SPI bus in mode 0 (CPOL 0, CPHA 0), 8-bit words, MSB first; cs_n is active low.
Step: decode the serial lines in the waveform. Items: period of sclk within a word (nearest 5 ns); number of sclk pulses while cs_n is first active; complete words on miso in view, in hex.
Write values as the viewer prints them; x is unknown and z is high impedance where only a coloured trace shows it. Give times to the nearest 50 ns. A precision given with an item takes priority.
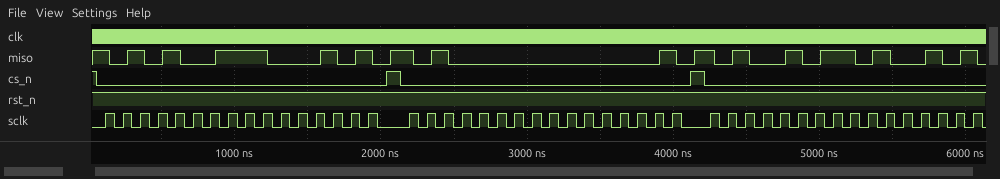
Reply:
120 ns
16
A9, C5, A0, 01, A5, A5
